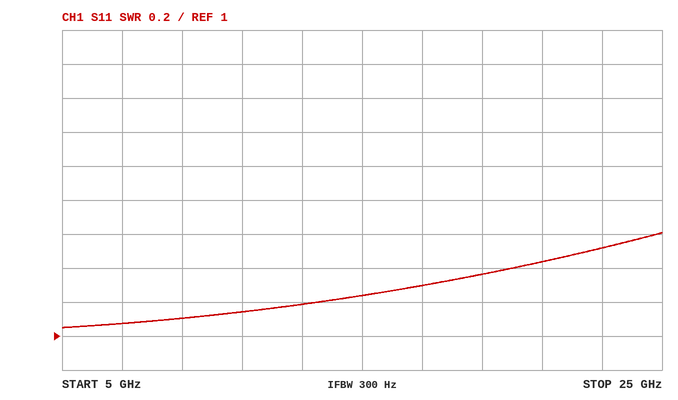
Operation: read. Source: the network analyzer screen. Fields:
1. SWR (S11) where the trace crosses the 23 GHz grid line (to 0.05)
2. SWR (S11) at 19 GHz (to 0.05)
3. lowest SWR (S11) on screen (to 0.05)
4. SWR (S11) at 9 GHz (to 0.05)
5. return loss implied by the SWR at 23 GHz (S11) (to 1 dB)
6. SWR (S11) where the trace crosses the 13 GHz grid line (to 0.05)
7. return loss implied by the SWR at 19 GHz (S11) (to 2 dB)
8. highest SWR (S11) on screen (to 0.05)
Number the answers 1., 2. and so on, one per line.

1. 1.50
2. 1.35
3. 1.05
4. 1.10
5. 14 dB
6. 1.20
7. 16 dB
8. 1.60
